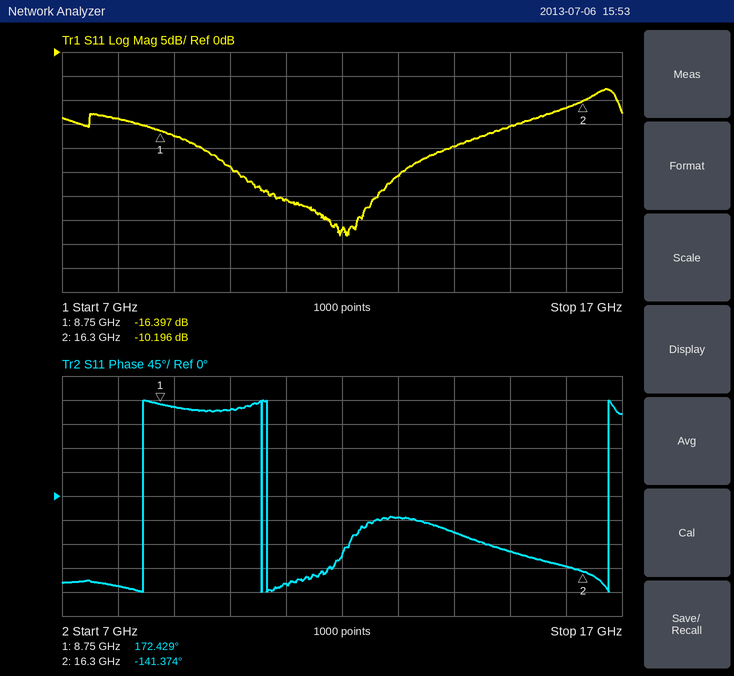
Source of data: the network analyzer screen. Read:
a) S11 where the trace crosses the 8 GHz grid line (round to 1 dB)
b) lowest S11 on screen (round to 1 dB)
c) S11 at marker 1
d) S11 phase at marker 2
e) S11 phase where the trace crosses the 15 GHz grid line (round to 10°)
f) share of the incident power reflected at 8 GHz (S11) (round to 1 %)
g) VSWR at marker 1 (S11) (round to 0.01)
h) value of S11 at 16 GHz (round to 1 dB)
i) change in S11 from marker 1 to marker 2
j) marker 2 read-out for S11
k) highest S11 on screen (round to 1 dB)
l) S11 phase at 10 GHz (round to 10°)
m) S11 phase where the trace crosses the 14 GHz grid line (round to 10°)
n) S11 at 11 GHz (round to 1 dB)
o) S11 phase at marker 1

-14 dB
-38 dB
-16.397 dB
-141.374°
-100°
4 %
1.36
-12 dB
6.201 dB
-10.196 dB
-8 dB
160°
-70°
-31 dB
172.429°
